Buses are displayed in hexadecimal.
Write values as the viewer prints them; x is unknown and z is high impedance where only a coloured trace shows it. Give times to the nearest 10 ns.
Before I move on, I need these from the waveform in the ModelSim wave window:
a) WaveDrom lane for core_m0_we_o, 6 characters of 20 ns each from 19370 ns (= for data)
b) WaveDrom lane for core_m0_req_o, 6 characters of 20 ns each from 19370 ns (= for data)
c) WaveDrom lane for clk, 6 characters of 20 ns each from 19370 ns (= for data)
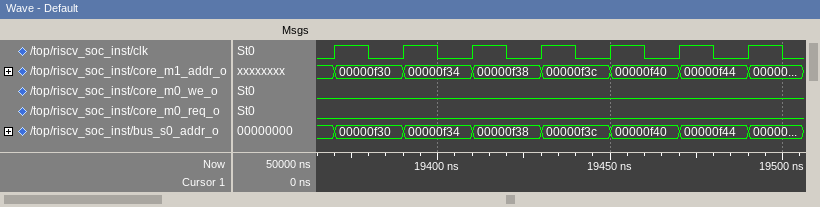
{name: 'core_m0_we_o', wave: '0.....'}
{name: 'core_m0_req_o', wave: '0.....'}
{name: 'clk', wave: 'p.....'}
